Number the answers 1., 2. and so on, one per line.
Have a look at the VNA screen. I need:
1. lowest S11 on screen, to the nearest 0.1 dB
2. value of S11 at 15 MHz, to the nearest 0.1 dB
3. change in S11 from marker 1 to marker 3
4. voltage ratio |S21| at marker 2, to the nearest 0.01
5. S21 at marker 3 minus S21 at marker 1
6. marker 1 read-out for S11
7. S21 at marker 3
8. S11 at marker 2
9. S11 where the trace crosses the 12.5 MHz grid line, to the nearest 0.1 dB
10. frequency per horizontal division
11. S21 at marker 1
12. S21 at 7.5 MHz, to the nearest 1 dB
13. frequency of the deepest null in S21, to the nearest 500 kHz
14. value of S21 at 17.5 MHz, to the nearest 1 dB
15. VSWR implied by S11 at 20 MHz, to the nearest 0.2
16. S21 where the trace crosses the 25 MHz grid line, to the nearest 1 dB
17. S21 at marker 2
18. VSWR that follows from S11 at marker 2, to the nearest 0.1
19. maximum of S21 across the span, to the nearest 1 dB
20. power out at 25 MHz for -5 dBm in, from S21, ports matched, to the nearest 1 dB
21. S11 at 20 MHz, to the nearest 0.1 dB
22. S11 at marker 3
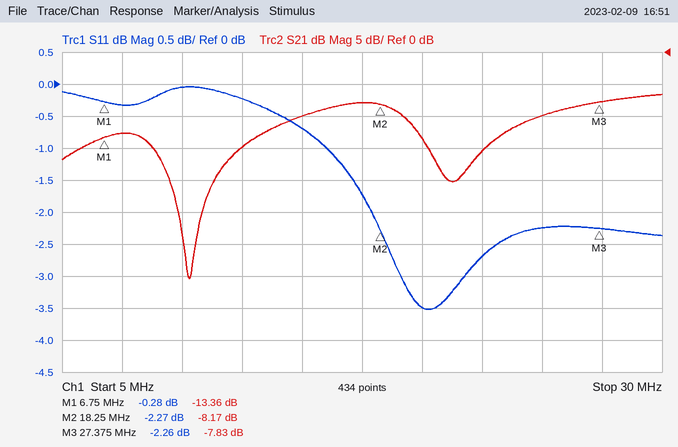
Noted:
1. -3.5 dB
2. -0.7 dB
3. -1.98 dB
4. 0.39
5. 5.53 dB
6. -0.28 dB
7. -7.83 dB
8. -2.27 dB
9. -0.2 dB
10. 2.5 MHz
11. -13.36 dB
12. -13 dB
13. 10.5 MHz
14. -8 dB
15. 5.0
16. -10 dB
17. -8.17 dB
18. 7.7
19. -7 dB
20. -15 dBm
21. -3.5 dB
22. -2.26 dB
